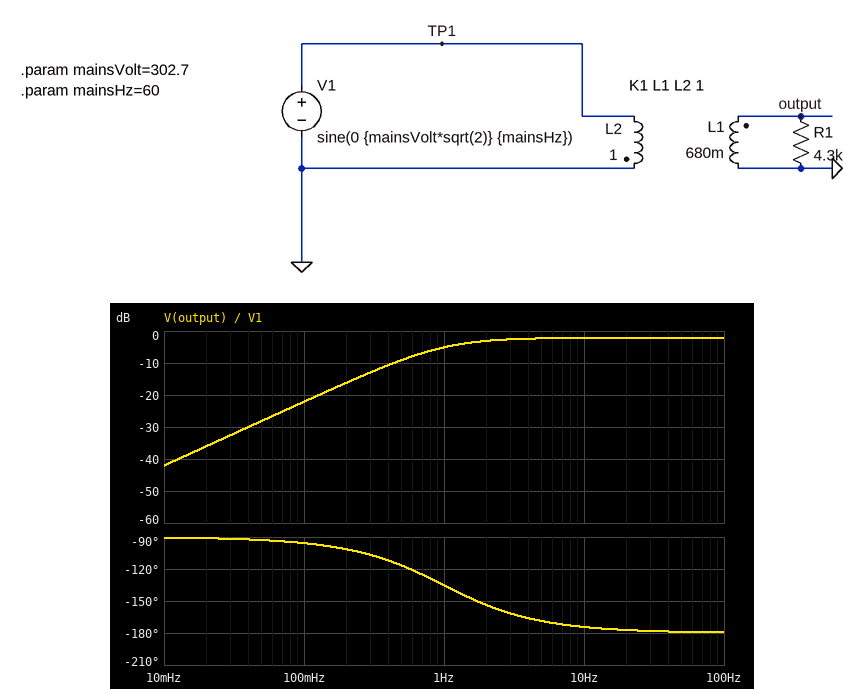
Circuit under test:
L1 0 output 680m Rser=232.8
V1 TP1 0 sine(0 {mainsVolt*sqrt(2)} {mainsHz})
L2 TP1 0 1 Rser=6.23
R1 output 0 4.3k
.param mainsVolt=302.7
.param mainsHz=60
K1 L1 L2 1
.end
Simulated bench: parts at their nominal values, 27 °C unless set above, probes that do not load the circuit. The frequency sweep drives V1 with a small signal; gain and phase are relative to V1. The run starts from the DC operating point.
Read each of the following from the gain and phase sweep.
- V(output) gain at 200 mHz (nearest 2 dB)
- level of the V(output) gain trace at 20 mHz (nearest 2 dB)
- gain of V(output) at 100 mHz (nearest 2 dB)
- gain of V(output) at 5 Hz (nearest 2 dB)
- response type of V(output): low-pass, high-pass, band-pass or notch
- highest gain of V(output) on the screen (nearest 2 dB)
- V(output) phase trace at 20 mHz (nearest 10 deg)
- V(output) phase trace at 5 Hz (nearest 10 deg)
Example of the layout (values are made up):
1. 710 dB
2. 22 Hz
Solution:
1. -16 dB
2. -36 dB
3. -22 dB
4. -2 dB
5. high-pass
6. -2 dB
7. -90 deg
8. -170 deg
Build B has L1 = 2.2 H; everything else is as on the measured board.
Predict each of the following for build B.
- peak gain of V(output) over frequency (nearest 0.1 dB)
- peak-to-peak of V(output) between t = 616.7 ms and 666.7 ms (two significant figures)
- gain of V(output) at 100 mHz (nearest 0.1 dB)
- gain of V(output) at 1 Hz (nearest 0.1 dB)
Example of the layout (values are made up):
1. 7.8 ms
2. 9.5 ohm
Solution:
1. 2.9 dB
2. 1.2 kV
3. -17.0 dB
4. 0 dB
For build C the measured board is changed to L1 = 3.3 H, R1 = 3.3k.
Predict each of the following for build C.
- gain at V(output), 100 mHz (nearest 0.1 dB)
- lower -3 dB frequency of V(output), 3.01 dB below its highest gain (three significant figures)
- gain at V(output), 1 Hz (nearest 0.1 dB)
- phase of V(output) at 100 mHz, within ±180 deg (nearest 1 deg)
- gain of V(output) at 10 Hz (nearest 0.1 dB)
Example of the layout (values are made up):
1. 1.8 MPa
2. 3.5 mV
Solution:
1. -15.4 dB
2. 986 mHz
3. 1.6 dB
4. -96 deg
5. 4.5 dB
